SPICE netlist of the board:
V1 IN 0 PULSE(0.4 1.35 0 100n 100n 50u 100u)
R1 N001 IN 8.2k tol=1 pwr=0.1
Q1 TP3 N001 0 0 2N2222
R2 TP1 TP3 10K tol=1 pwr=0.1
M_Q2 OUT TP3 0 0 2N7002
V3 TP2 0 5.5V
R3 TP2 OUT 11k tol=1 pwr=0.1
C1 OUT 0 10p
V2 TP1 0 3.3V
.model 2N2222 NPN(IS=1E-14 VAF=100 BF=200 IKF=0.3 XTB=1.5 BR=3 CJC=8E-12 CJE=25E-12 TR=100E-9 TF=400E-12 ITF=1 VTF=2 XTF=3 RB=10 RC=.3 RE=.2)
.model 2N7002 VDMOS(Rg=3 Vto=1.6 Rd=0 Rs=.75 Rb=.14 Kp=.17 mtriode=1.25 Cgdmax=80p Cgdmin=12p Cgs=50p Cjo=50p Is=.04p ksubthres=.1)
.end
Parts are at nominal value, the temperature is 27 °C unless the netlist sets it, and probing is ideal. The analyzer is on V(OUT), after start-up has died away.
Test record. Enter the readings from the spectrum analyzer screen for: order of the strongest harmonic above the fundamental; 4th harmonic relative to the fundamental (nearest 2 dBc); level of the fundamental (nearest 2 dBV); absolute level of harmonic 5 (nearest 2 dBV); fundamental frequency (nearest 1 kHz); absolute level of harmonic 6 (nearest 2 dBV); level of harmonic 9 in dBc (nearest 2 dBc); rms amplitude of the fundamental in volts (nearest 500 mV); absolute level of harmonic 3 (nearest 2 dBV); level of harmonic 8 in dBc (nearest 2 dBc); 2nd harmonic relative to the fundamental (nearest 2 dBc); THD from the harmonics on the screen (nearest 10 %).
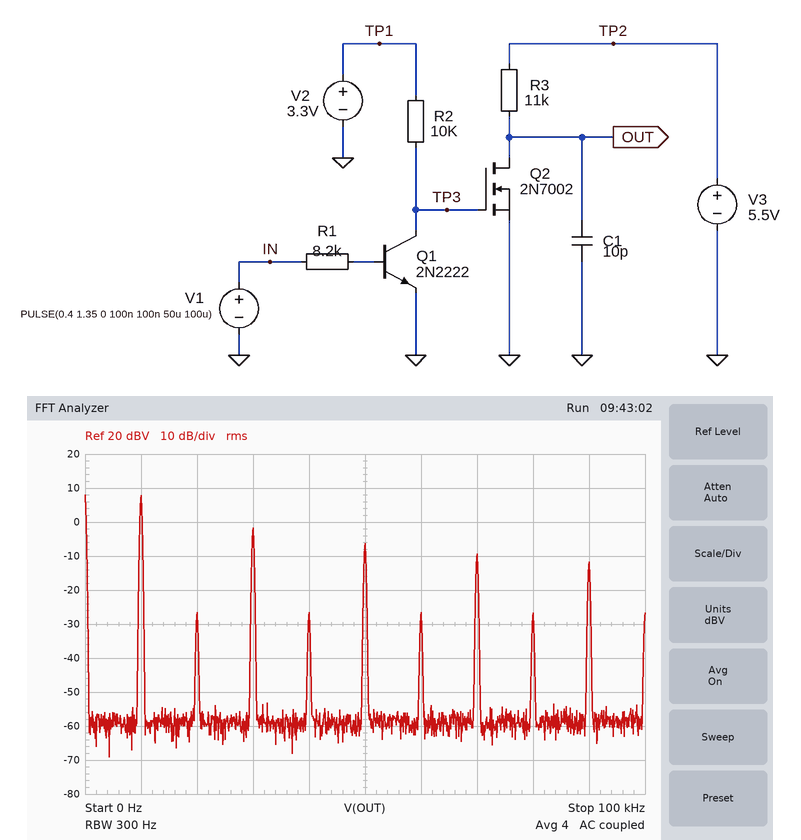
3
-34 dBc
8 dBV
-6 dBV
10 kHz
-26 dBV
-20 dBc
2.5 V
-2 dBV
-34 dBc
-34 dBc
40 %
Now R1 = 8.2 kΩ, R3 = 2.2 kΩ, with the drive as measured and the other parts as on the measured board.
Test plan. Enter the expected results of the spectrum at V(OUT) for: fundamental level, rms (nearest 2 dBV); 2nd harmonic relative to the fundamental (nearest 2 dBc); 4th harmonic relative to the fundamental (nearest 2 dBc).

8 dBV
-28 dBc
-28 dBc
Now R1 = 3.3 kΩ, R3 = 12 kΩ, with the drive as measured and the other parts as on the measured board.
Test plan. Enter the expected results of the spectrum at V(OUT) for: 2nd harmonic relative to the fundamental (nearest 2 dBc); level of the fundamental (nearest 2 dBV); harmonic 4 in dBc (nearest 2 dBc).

-36 dBc
8 dBV
-36 dBc
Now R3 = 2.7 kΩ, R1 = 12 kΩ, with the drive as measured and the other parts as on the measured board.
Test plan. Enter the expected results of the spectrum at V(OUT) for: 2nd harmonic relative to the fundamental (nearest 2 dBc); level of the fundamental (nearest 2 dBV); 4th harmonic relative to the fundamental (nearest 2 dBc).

-28 dBc
8 dBV
-28 dBc
